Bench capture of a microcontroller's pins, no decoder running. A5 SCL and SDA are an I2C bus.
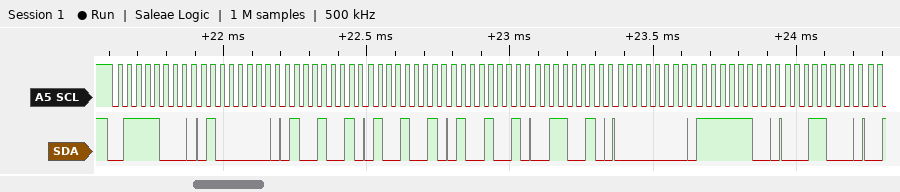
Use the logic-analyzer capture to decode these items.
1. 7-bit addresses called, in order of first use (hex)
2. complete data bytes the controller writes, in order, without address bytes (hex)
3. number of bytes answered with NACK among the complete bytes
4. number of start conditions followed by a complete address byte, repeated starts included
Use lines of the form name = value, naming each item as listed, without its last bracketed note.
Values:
7-bit addresses called, in order of first use = 0x3C
complete data bytes the controller writes, in order, without address bytes = 40 49 49 49 32 00 FC 18
number of bytes answered with NACK among the complete bytes = 0
number of start conditions followed by a complete address byte, repeated starts included = 1
